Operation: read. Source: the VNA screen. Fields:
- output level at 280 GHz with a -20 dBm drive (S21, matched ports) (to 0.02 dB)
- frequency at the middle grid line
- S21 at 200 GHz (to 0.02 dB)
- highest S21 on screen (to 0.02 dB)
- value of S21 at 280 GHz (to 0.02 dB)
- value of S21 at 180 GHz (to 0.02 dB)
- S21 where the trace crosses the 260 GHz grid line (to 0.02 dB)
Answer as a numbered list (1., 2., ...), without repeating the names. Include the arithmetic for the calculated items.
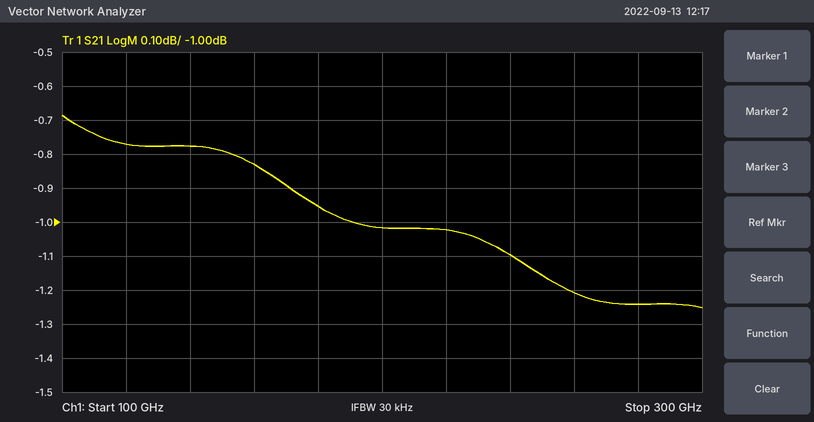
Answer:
1. -20 dBm + (-1.24 dB) = -21.24 dBm
2. 200 GHz
3. -1.02 dB
4. -0.68 dB
5. -1.24 dB
6. -0.96 dB
7. -1.20 dB
